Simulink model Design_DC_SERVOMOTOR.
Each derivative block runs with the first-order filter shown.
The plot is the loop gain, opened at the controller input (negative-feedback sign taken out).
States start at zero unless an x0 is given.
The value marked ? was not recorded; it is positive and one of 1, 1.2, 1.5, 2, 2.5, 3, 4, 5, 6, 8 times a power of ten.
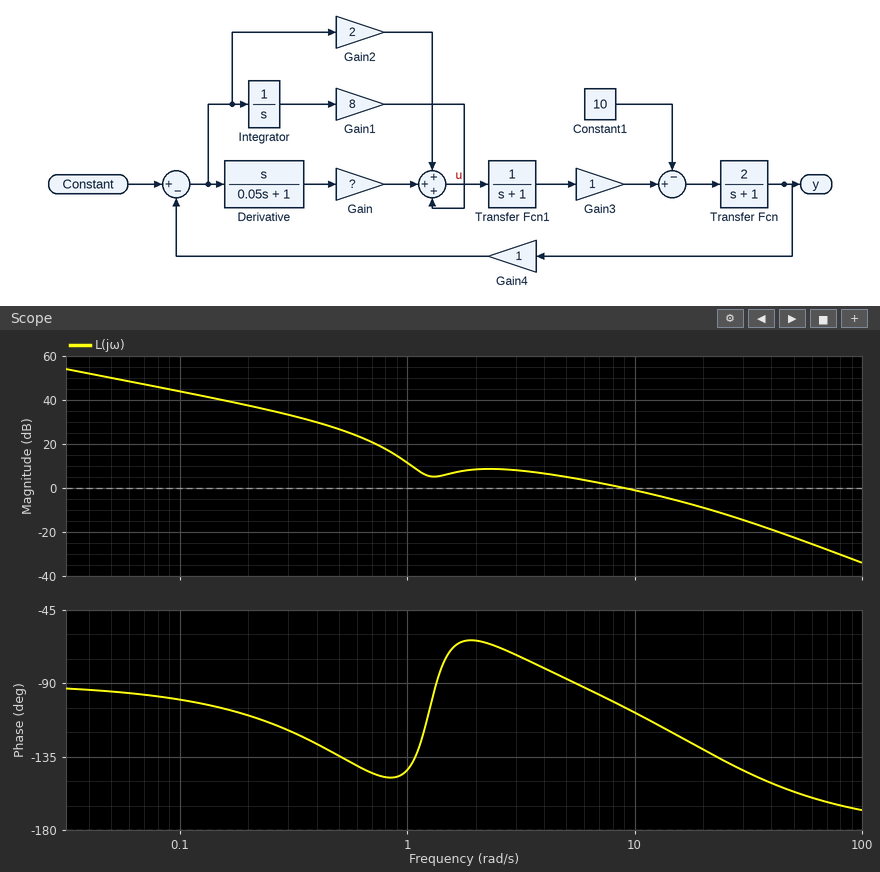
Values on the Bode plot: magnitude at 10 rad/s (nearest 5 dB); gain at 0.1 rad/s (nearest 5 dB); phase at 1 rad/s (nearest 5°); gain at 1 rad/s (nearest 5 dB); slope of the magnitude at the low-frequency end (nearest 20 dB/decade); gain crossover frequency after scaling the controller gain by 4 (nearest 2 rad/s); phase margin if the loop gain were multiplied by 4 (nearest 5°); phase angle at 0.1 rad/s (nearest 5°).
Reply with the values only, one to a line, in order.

0 dB
45 dB
-145°
10 dB
-20 dB/decade
26 rad/s
40°
-100°
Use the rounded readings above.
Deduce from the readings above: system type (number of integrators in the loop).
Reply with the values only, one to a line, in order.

1
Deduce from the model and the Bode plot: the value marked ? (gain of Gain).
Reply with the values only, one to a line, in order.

5
